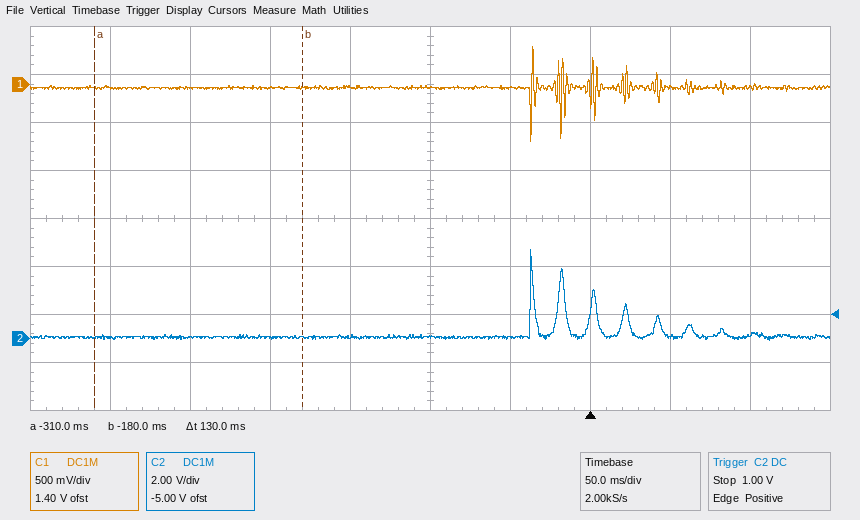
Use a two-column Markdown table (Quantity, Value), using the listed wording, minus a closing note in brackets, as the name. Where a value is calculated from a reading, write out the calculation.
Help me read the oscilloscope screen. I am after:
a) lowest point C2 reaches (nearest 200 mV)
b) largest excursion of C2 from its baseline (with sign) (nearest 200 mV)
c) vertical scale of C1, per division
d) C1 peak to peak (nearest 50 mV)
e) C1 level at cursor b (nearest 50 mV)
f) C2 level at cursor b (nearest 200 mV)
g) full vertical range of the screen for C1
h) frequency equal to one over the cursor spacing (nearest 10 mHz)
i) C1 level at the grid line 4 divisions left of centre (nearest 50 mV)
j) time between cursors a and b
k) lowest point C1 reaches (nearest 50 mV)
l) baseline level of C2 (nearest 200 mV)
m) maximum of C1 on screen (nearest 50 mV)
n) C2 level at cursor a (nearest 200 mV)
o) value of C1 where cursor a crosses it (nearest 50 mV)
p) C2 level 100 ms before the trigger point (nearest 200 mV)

| Quantity | Value |
|---|---|
| lowest point C2 reaches | 0.0 V |
| largest excursion of C2 from its baseline (with sign) | +3.6 V |
| vertical scale of C1, per division | 500 mV |
| C1 peak to peak | 400 mV − (-600 mV) = 1.00 V |
| C1 level at cursor b | -50 mV |
| C2 level at cursor b | 0.0 V |
| full vertical range of the screen for C1 | 4 V |
| frequency equal to one over the cursor spacing | 1 / 130 ms ≈ 7.69 Hz |
| C1 level at the grid line 4 divisions left of centre | -50 mV |
| time between cursors a and b | 130 ms |
| lowest point C1 reaches | -600 mV |
| baseline level of C2 | 0.0 V |
| maximum of C1 on screen | 400 mV |
| C2 level at cursor a | 0.0 V |
| value of C1 where cursor a crosses it | -50 mV |
| C2 level 100 ms before the trigger point | 0.0 V |
